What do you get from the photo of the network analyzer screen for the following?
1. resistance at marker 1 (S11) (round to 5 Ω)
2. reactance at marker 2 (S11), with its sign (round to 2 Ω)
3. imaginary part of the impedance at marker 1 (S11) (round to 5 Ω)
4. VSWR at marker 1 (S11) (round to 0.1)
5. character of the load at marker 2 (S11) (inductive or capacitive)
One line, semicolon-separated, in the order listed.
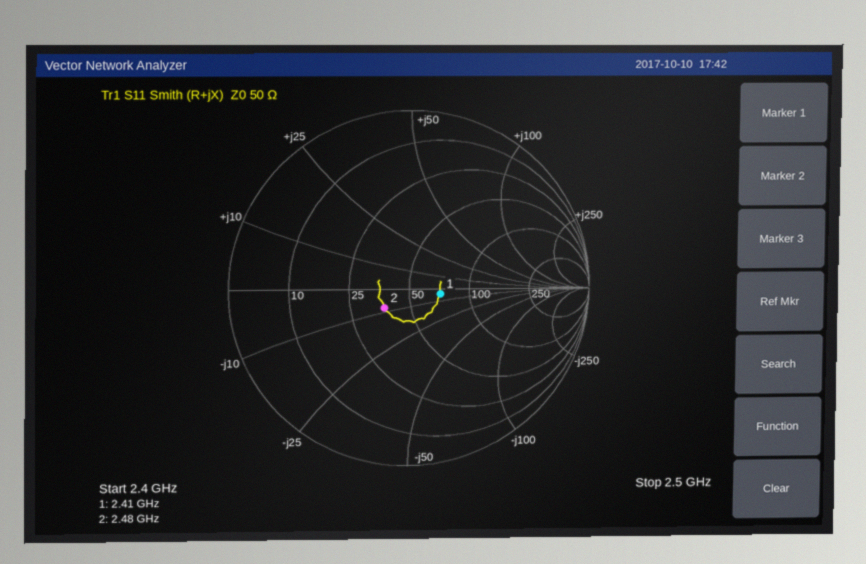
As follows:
70 Ω; -8 Ω; -5 Ω; 1.4; capacitive
